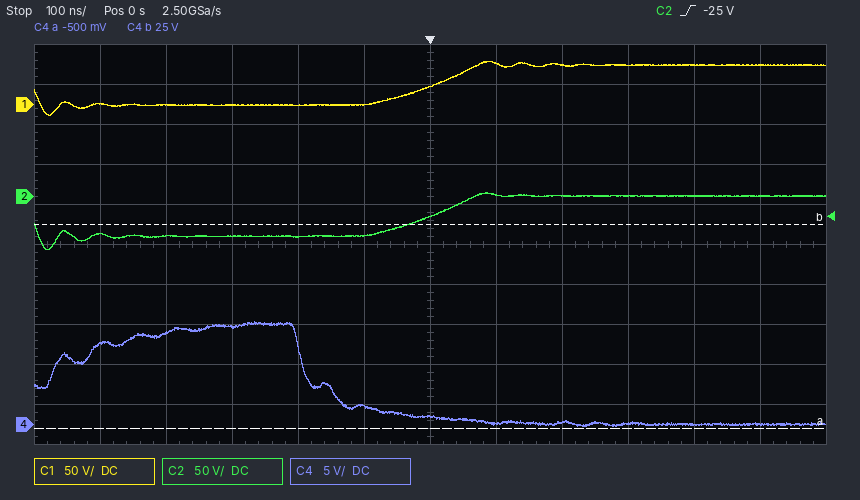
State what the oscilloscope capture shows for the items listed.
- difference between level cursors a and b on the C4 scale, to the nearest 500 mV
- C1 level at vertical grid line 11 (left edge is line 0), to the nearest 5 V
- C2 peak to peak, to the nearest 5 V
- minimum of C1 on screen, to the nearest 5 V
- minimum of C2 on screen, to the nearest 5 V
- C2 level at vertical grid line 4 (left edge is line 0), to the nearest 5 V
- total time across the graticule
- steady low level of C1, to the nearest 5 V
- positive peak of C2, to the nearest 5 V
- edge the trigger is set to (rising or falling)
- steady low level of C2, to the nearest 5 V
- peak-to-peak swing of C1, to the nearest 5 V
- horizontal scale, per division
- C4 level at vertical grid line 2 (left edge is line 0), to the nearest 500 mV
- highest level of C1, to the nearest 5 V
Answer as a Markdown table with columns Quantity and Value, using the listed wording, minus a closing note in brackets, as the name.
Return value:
| Quantity | Value |
|---|---|
| difference between level cursors a and b on the C4 scale, to the nearest 500 mV | 25.5 V |
| C1 level at vertical grid line 11 (left edge is line 0), to the nearest 5 V | 50 V |
| C2 peak to peak, to the nearest 5 V | 70 V |
| minimum of C1 on screen, to the nearest 5 V | -15 V |
| minimum of C2 on screen, to the nearest 5 V | -65 V |
| C2 level at vertical grid line 4 (left edge is line 0), to the nearest 5 V | -50 V |
| total time across the graticule | 1.2 µs |
| steady low level of C1, to the nearest 5 V | 0 V |
| positive peak of C2, to the nearest 5 V | 5 V |
| edge the trigger is set to | rising |
| steady low level of C2, to the nearest 5 V | -50 V |
| peak-to-peak swing of C1, to the nearest 5 V | 70 V |
| horizontal scale, per division | 100 ns |
| C4 level at vertical grid line 2 (left edge is line 0), to the nearest 500 mV | 11.5 V |
| highest level of C1, to the nearest 5 V | 55 V |
